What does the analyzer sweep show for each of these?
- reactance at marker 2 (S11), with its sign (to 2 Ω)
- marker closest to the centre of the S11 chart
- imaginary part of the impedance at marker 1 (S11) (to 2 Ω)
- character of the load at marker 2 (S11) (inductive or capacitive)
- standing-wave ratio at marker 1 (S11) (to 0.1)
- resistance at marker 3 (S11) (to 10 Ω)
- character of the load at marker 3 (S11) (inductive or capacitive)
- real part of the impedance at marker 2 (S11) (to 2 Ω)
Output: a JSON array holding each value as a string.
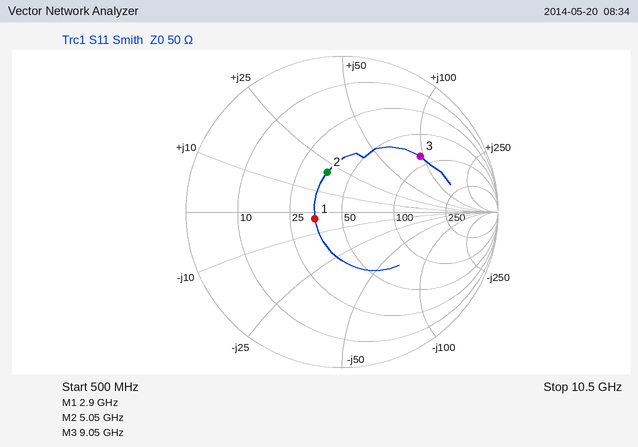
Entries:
["+20 Ω", "marker 1", "-4 Ω", "inductive", "1.4", "80 Ω", "inductive", "36 Ω"]
